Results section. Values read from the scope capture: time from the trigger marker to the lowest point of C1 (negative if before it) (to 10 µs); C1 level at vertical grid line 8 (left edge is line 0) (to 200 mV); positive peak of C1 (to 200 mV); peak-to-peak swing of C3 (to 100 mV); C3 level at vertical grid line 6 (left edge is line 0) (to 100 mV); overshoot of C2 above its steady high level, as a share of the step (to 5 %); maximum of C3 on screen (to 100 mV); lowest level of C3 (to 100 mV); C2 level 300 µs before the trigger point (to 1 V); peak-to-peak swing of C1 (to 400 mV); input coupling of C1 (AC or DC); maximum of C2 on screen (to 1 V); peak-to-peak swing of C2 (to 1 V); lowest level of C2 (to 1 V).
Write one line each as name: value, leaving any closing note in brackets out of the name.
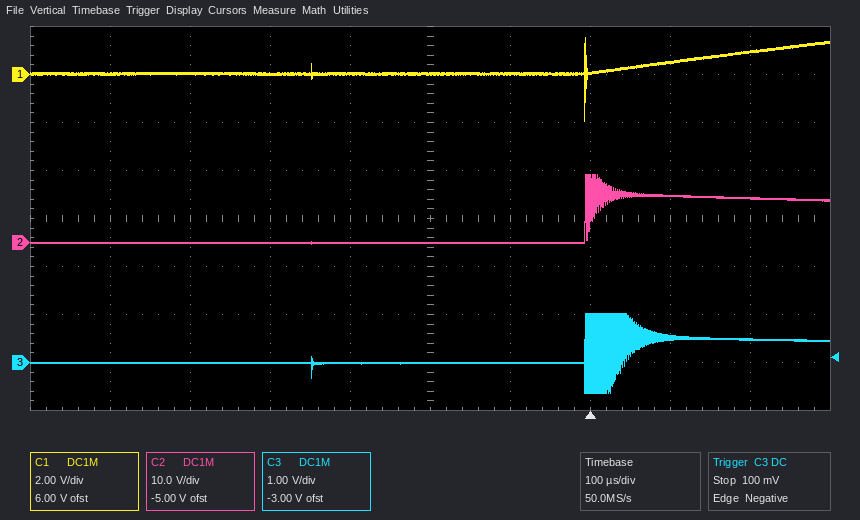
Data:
time from the trigger marker to the lowest point of C1 (negative if before it): -10 µs
C1 level at vertical grid line 8 (left edge is line 0): 600 mV
positive peak of C1: 1.6 V
peak-to-peak swing of C3: 1.6 V
C3 level at vertical grid line 6 (left edge is line 0): 0.0 V
overshoot of C2 above its steady high level, as a share of the step: 50 %
maximum of C3 on screen: 1.0 V
lowest level of C3: -600 mV
C2 level 300 µs before the trigger point: 0 V
peak-to-peak swing of C1: 3.6 V
input coupling of C1: DC
maximum of C2 on screen: 14 V
peak-to-peak swing of C2: 14 V
lowest level of C2: 0 V
